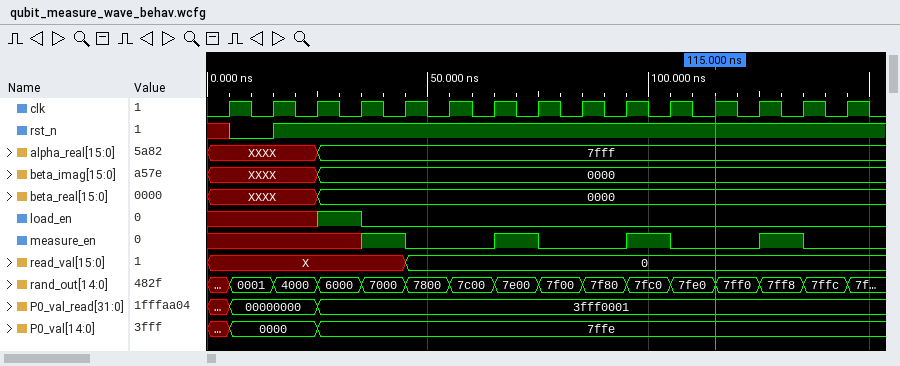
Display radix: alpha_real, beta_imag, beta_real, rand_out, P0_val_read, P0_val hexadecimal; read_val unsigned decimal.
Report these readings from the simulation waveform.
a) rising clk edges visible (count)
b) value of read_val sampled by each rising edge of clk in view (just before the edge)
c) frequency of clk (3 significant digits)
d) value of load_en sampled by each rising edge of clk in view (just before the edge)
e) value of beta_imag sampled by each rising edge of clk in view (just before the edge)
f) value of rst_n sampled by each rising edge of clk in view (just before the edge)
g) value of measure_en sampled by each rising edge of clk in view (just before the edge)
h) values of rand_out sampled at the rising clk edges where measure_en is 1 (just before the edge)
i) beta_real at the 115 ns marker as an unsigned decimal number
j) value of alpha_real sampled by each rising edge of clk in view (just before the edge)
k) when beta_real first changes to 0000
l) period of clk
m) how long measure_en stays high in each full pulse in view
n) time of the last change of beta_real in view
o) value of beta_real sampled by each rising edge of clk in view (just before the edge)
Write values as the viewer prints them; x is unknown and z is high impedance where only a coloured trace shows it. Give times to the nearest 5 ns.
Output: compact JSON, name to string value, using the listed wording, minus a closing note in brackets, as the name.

{"rising clk edges visible": "15", "value of read_val sampled by each rising edge of clk in view": "X, X, X, X, X, 0, 0, 0, 0, 0, 0, 0, 0, 0, 0", "frequency of clk": "100 MHz", "value of load_en sampled by each rising edge of clk in view": "x x x 1 0 0 0 0 0 0 0 0 0 0 0", "value of beta_imag sampled by each rising edge of clk in view": "XXXX, XXXX, XXXX, 0000, 0000, 0000, 0000, 0000, 0000, 0000, 0000, 0000, 0000, 0000, 0000", "value of rst_n sampled by each rising edge of clk in view": "x 0 1 1 1 1 1 1 1 1 1 1 1 1 1", "value of measure_en sampled by each rising edge of clk in view": "x x x x 1 0 0 1 0 0 1 0 0 1 0", "values of rand_out sampled at the rising clk edges where measure_en is 1": "7000, 7e00, 7fc0, 7ff8", "beta_real at the 115 ns marker as an unsigned decimal number": "0", "value of alpha_real sampled by each rising edge of clk in view": "XXXX, XXXX, XXXX, 7fff, 7fff, 7fff, 7fff, 7fff, 7fff, 7fff, 7fff, 7fff, 7fff, 7fff, 7fff", "when beta_real first changes to 0000": "25 ns", "period of clk": "10 ns", "how long measure_en stays high in each full pulse in view": "10 ns, 10 ns, 10 ns", "time of the last change of beta_real in view": "25 ns", "value of beta_real sampled by each rising edge of clk in view": "XXXX, XXXX, XXXX, 0000, 0000, 0000, 0000, 0000, 0000, 0000, 0000, 0000, 0000, 0000, 0000"}
